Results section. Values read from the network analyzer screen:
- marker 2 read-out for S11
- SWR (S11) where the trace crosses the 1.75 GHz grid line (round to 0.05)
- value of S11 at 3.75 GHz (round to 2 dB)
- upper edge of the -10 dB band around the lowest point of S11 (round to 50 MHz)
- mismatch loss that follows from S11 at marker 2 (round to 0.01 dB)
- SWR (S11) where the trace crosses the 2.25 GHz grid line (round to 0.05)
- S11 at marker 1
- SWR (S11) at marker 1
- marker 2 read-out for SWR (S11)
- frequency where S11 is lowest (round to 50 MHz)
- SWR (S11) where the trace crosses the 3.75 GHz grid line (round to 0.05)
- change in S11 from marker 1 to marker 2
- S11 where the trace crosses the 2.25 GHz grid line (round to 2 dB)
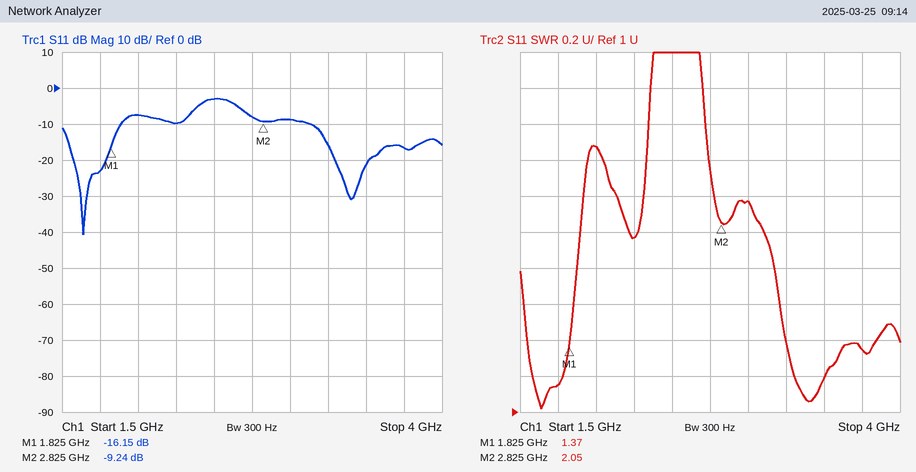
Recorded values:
-9.24 dB
1.15
-16 dB
1.90 GHz
0.55 dB
1.95
-16.15 dB
1.37
2.05
1.65 GHz
1.35
6.91 dB
-10 dB
